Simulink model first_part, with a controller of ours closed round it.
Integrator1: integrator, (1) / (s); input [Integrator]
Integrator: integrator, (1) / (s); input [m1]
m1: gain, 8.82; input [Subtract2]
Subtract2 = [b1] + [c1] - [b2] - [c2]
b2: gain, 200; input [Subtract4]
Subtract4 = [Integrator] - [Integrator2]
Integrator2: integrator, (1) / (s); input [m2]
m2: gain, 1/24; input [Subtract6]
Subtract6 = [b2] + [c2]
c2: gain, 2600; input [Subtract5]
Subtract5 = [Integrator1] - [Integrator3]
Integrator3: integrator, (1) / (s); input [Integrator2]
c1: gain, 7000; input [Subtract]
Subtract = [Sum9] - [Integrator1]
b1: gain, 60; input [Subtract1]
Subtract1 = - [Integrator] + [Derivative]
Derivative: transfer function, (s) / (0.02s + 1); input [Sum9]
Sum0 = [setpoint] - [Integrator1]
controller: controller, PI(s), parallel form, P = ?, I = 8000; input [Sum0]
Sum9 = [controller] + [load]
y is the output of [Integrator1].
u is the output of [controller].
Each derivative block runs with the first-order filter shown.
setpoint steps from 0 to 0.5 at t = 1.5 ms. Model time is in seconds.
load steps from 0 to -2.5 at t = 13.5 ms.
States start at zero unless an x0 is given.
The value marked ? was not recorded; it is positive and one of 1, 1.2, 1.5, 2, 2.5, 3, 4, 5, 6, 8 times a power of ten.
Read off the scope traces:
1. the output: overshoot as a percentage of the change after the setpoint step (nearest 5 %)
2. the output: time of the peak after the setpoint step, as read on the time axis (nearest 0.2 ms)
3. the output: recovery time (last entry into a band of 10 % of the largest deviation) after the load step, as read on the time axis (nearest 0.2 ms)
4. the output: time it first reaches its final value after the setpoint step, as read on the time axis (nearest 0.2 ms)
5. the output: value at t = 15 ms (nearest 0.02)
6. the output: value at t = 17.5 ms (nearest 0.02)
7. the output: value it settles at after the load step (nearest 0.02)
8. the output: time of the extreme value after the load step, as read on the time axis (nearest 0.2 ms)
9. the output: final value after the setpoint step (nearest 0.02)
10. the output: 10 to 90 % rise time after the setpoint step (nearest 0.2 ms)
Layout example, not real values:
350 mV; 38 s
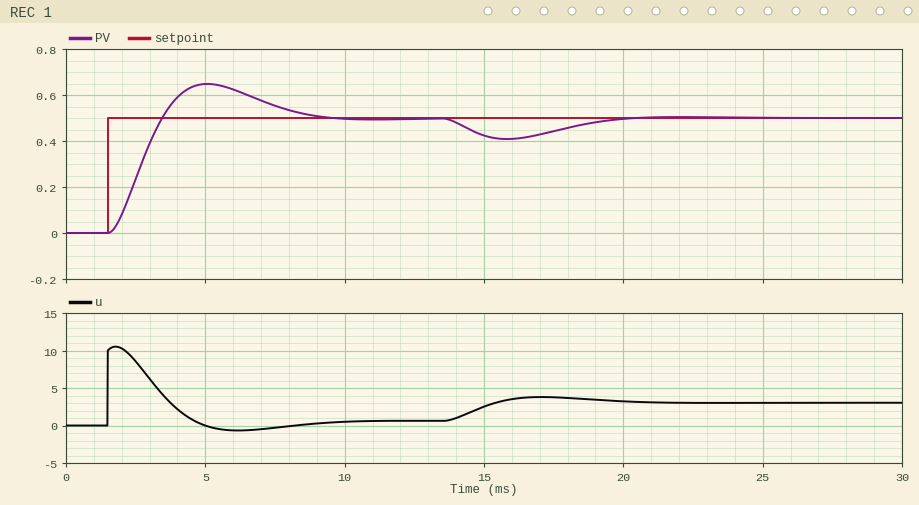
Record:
30 %; 5.0 ms; 19.6 ms; 3.4 ms; 0.42; 0.44; 0.50; 15.8 ms; 0.50; 1.4 ms
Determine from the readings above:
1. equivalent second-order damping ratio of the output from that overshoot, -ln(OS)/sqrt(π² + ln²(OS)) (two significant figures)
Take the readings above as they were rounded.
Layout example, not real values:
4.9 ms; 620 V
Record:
0.36
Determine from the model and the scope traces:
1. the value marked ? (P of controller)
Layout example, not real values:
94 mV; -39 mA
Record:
20
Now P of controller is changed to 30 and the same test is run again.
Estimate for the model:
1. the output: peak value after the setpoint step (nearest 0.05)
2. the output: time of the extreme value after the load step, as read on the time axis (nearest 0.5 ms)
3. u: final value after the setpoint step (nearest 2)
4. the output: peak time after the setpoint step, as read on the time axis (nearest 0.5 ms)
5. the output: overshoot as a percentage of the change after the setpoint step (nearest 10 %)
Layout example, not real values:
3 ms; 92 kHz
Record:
0.60; 15.5 ms; 0; 4.0 ms; 20 %
